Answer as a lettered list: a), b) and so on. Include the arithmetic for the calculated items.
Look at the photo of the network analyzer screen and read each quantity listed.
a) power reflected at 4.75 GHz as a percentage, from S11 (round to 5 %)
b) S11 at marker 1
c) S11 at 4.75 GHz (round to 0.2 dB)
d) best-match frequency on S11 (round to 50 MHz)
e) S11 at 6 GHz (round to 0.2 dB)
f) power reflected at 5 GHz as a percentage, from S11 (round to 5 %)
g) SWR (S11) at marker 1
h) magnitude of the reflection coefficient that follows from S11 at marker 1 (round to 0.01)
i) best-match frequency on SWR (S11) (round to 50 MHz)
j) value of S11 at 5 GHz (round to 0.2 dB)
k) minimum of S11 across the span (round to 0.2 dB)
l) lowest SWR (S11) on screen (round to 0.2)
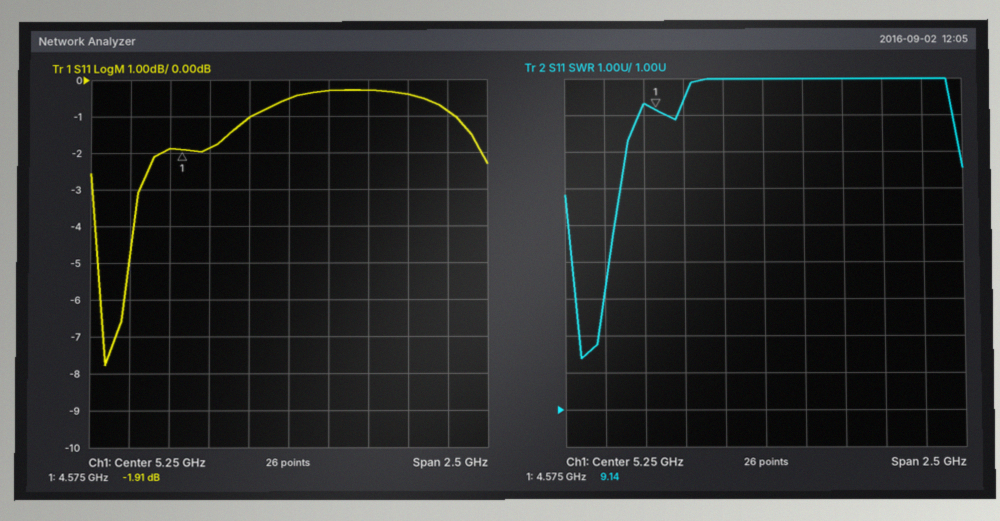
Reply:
a) 10^(-1.8/10) ≈ 66.1 %, so 65 % to the nearest 5 %
b) -1.91 dB
c) -1.8 dB
d) 4.10 GHz
e) -0.4 dB
f) 10^(-1/10) ≈ 79.4 %, so 80 % to the nearest 5 %
g) 9.14
h) 10^(-1.91/20) ≈ 0.80
i) 4.10 GHz
j) -1.0 dB
k) -7.8 dB
l) 2.4
